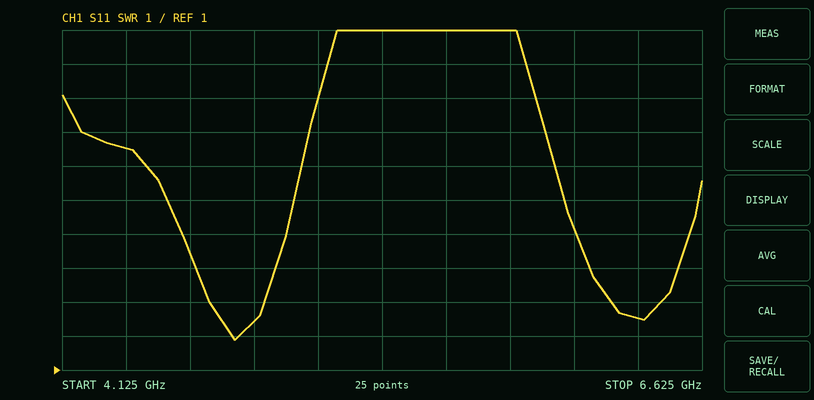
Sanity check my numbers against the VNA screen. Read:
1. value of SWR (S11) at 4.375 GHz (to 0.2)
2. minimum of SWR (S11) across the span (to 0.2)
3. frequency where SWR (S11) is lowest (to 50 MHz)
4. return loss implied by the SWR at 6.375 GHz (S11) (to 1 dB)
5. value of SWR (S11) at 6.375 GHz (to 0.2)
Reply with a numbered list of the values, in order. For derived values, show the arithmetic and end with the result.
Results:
1. 7.6
2. 1.8
3. 4.80 GHz
4. −20 log10((2.6 − 1)/(2.6 + 1)) ≈ 7 dB
5. 2.6
